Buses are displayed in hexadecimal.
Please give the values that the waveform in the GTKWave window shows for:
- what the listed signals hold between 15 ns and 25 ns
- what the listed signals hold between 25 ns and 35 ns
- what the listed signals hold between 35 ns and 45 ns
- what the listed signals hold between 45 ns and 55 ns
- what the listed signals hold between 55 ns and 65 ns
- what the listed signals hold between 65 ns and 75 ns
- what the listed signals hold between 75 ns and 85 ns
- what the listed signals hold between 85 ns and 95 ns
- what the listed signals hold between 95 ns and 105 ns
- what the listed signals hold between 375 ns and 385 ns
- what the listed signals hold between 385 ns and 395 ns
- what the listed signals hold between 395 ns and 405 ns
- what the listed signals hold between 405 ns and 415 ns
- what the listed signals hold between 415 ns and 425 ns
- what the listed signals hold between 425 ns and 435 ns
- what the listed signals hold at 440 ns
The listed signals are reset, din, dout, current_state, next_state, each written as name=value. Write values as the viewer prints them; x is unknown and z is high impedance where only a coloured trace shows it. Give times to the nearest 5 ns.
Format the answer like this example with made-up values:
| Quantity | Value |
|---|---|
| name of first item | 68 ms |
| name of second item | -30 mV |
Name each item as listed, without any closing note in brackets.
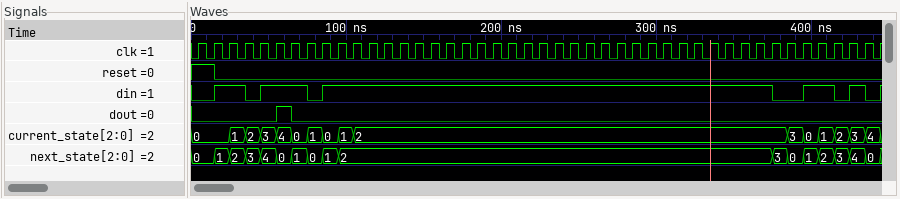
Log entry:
| Quantity | Value |
|---|---|
| what the listed signals hold between 15 ns and 25 ns | reset=0, din=1, dout=0, current_state=0, next_state=1 |
| what the listed signals hold between 25 ns and 35 ns | reset=0, din=1, dout=0, current_state=1, next_state=2 |
| what the listed signals hold between 35 ns and 45 ns | reset=0, din=0, dout=0, current_state=2, next_state=3 |
| what the listed signals hold between 45 ns and 55 ns | reset=0, din=1, dout=0, current_state=3, next_state=4 |
| what the listed signals hold between 55 ns and 65 ns | reset=0, din=1, dout=1, current_state=4, next_state=0 |
| what the listed signals hold between 65 ns and 75 ns | reset=0, din=1, dout=0, current_state=0, next_state=1 |
| what the listed signals hold between 75 ns and 85 ns | reset=0, din=0, dout=0, current_state=1, next_state=0 |
| what the listed signals hold between 85 ns and 95 ns | reset=0, din=1, dout=0, current_state=0, next_state=1 |
| what the listed signals hold between 95 ns and 105 ns | reset=0, din=1, dout=0, current_state=1, next_state=2 |
| what the listed signals hold between 375 ns and 385 ns | reset=0, din=0, dout=0, current_state=2, next_state=3 |
| what the listed signals hold between 385 ns and 395 ns | reset=0, din=0, dout=0, current_state=3, next_state=0 |
| what the listed signals hold between 395 ns and 405 ns | reset=0, din=1, dout=0, current_state=0, next_state=1 |
| what the listed signals hold between 405 ns and 415 ns | reset=0, din=1, dout=0, current_state=1, next_state=2 |
| what the listed signals hold between 415 ns and 425 ns | reset=0, din=0, dout=0, current_state=2, next_state=3 |
| what the listed signals hold between 425 ns and 435 ns | reset=0, din=1, dout=0, current_state=3, next_state=4 |
| what the listed signals hold at 440 ns | reset=0, din=0, dout=0, current_state=4, next_state=0 |
